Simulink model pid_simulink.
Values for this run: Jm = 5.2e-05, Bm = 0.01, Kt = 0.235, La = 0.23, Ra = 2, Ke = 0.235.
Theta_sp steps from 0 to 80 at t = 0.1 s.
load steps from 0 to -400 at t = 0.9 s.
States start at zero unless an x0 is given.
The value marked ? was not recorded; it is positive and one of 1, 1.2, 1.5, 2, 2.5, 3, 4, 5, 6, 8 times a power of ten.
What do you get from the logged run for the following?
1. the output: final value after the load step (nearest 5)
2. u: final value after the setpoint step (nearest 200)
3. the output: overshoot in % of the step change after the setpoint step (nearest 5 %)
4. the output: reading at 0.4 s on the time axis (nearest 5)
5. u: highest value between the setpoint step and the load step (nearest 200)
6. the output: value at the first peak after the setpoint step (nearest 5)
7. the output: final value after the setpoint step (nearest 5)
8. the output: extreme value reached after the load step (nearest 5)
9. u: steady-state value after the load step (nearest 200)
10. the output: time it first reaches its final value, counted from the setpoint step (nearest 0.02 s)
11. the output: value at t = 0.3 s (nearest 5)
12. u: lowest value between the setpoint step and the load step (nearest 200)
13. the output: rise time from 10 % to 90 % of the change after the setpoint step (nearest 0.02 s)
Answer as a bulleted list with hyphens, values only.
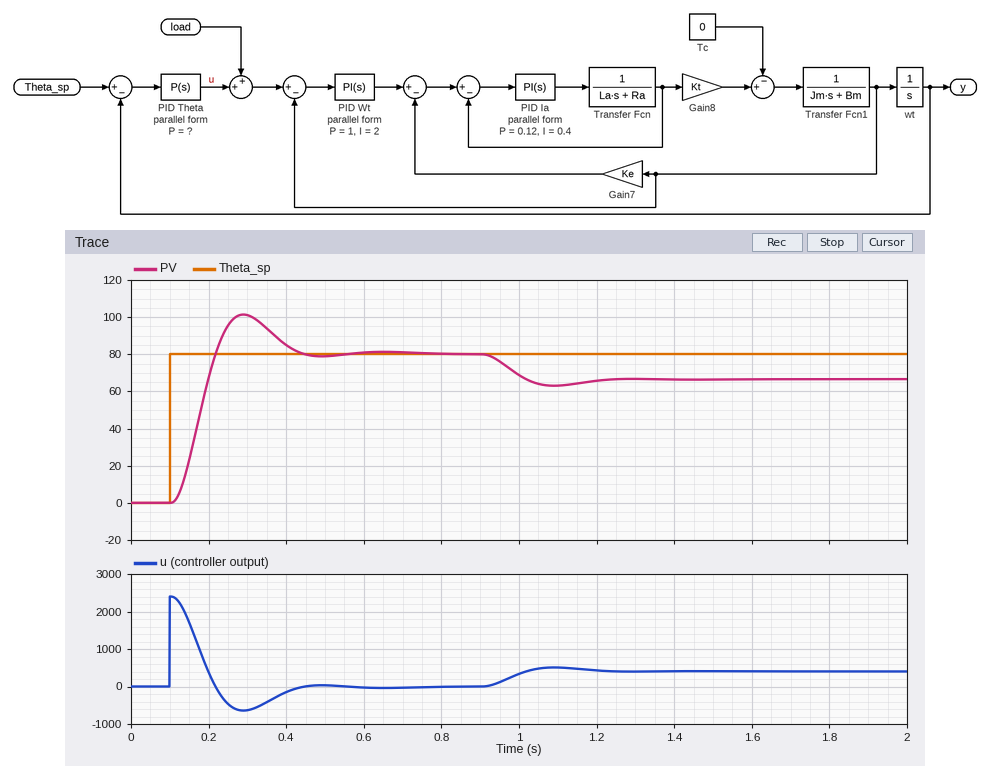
- 65
- 0
- 25 %
- 85
- 2400
- 100
- 80
- 65
- 400
- 0.12 s
- 100
- -600
- 0.08 s
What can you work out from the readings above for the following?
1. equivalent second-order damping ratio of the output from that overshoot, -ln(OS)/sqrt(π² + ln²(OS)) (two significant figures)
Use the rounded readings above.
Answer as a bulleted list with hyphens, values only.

- 0.40
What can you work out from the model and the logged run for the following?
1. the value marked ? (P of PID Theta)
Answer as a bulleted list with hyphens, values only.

- 30
